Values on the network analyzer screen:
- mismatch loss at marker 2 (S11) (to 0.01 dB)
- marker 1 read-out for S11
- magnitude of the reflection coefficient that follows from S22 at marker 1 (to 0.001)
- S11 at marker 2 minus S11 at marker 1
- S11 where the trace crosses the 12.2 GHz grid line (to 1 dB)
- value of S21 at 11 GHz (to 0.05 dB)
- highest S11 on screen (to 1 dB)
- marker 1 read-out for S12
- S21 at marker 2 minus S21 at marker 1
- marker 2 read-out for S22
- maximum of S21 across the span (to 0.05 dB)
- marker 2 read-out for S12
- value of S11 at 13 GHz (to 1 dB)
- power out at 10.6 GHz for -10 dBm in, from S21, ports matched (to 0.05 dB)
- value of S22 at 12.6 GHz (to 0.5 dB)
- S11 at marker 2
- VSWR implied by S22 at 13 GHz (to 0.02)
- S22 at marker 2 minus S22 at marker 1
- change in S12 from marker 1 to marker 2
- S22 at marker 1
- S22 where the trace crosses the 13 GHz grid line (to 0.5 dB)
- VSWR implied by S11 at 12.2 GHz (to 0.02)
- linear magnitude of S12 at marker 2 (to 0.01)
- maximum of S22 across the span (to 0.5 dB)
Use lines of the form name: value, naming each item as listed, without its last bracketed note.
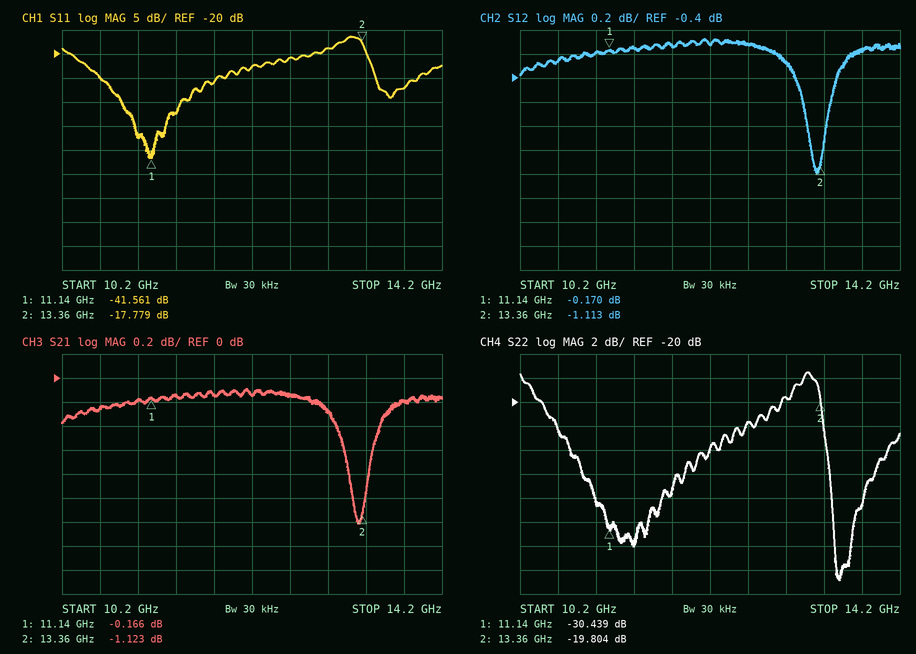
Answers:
mismatch loss at marker 2 (S11): 0.07 dB
marker 1 read-out for S11: -41.561 dB
magnitude of the reflection coefficient that follows from S22 at marker 1: 0.030
S11 at marker 2 minus S11 at marker 1: 23.782 dB
S11 where the trace crosses the 12.2 GHz grid line: -23 dB
value of S21 at 11 GHz: -0.20 dB
highest S11 on screen: -16 dB
marker 1 read-out for S12: -0.170 dB
S21 at marker 2 minus S21 at marker 1: -0.957 dB
marker 2 read-out for S22: -19.804 dB
maximum of S21 across the span: -0.10 dB
marker 2 read-out for S12: -1.113 dB
value of S11 at 13 GHz: -19 dB
power out at 10.6 GHz for -10 dBm in, from S21, ports matched: -10.25 dBm
value of S22 at 12.6 GHz: -21.5 dB
S11 at marker 2: -17.779 dB
VSWR implied by S22 at 13 GHz: 1.24
S22 at marker 2 minus S22 at marker 1: 10.635 dB
change in S12 from marker 1 to marker 2: -0.943 dB
S22 at marker 1: -30.439 dB
S22 where the trace crosses the 13 GHz grid line: -19.5 dB
VSWR implied by S11 at 12.2 GHz: 1.16
linear magnitude of S12 at marker 2: 0.88
maximum of S22 across the span: -17.5 dB
